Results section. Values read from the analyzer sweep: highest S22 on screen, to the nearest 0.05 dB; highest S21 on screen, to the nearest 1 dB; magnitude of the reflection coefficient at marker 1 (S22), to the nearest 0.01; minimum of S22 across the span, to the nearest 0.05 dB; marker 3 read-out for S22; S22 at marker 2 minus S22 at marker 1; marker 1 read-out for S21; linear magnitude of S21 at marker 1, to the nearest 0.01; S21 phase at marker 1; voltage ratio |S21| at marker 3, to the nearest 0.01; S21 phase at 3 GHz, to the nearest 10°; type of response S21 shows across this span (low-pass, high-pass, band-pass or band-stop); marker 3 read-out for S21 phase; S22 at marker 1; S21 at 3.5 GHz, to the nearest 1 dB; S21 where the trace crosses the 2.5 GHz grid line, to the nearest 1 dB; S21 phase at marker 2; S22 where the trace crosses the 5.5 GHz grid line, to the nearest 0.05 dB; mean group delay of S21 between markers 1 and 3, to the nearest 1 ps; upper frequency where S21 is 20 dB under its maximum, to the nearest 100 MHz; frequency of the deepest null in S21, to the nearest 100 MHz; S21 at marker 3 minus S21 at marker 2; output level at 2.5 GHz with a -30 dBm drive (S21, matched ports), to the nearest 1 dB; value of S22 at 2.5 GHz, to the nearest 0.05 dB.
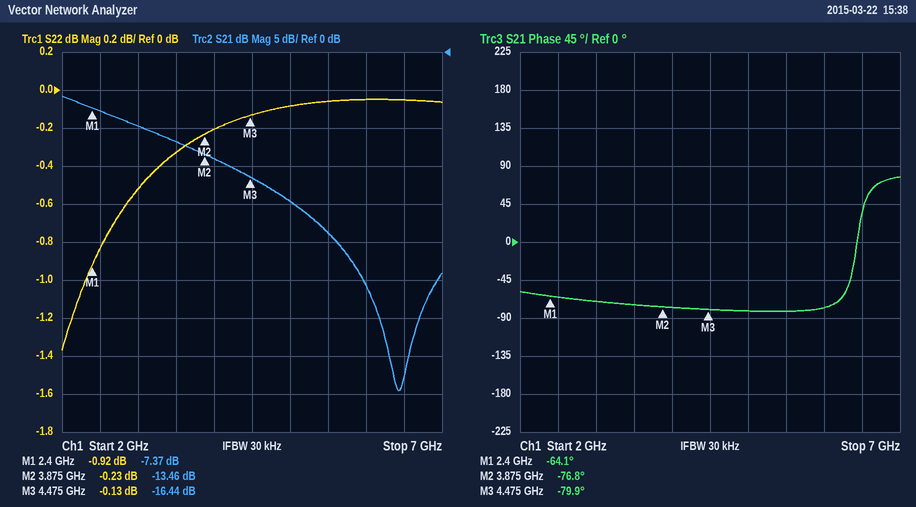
-0.05 dB
-6 dB
0.90
-1.35 dB
-0.13 dB
0.69 dB
-7.37 dB
0.43
-64.1°
0.15
-70°
low-pass
-79.9°
-0.92 dB
-12 dB
-8 dB
-76.8°
-0.05 dB
21 ps
5.7 GHz
6.4 GHz
-2.98 dB
-38 dBm
-0.85 dB
